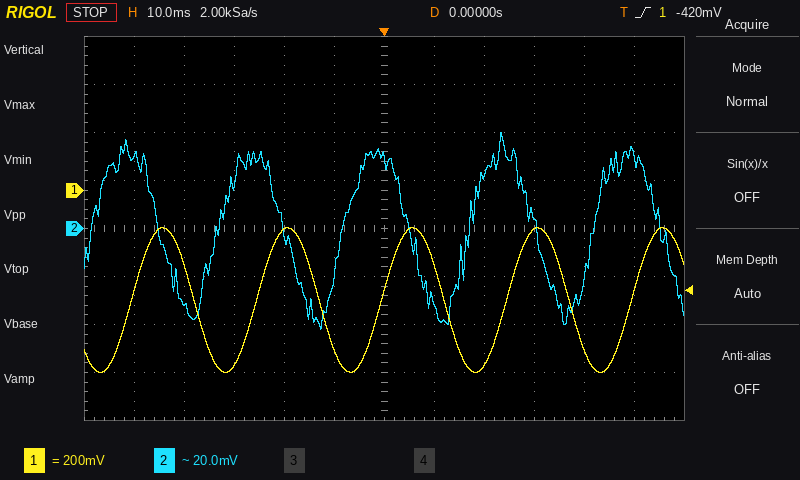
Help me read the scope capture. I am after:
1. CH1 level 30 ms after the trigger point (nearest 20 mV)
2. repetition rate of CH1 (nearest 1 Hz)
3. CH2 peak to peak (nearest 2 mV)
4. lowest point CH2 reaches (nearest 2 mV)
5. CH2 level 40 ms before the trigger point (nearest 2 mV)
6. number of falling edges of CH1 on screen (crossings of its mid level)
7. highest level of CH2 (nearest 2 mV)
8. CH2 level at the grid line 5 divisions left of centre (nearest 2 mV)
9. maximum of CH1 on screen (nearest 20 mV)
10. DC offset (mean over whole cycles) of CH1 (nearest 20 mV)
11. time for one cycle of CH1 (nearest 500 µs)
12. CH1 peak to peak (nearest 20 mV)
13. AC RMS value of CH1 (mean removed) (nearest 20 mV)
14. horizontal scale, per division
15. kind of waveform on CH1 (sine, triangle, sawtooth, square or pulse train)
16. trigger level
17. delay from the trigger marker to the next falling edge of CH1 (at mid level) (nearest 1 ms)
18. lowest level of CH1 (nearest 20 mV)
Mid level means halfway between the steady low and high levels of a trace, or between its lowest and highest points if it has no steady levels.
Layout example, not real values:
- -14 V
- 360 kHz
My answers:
- -160 mV
- 40 Hz
- 82 mV
- -42 mV
- -32 mV
- 4
- 40 mV
- 30 mV
- -160 mV
- -460 mV
- 25.0 ms
- 600 mV
- 220 mV
- 10 ms
- sine
- -420 mV
- 12 ms
- -760 mV
